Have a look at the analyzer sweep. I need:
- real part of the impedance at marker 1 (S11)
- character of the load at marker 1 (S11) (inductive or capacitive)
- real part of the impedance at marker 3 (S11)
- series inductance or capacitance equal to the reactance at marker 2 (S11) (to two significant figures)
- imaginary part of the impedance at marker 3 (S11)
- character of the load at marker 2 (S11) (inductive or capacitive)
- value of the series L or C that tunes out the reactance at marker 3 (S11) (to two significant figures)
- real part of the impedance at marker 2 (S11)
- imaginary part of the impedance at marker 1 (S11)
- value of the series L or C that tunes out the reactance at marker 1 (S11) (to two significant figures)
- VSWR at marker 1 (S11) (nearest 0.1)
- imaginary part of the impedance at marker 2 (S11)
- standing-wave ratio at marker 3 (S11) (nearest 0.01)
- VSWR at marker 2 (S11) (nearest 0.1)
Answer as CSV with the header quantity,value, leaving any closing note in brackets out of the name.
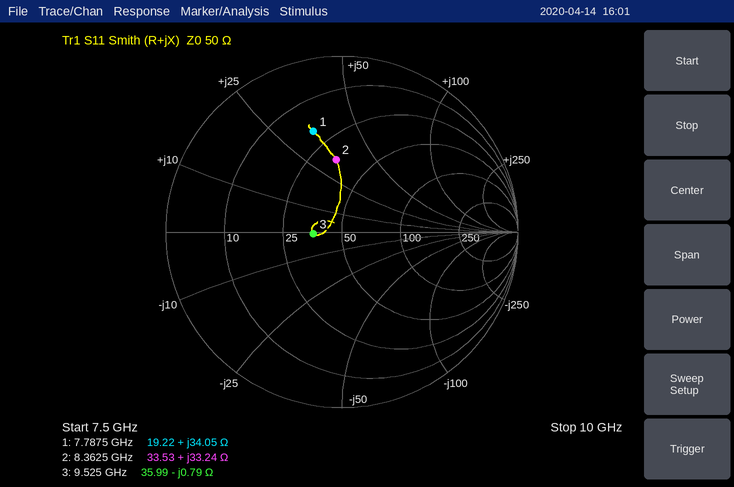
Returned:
quantity,value
real part of the impedance at marker 1,19.22 Ω
character of the load at marker 1 (S11),inductive
real part of the impedance at marker 3,35.99 Ω
series inductance or capacitance equal to the reactance at marker 2 (S11),630 pH
imaginary part of the impedance at marker 3,-0.79 Ω
character of the load at marker 2 (S11),inductive
value of the series L or C that tunes out the reactance at marker 3 (S11),13 pH
real part of the impedance at marker 2,33.53 Ω
imaginary part of the impedance at marker 1,+34.05 Ω
value of the series L or C that tunes out the reactance at marker 1 (S11),600 fF
VSWR at marker 1 (S11),3.9
imaginary part of the impedance at marker 2,+33.24 Ω
standing-wave ratio at marker 3 (S11),1.39
VSWR at marker 2 (S11),2.4
